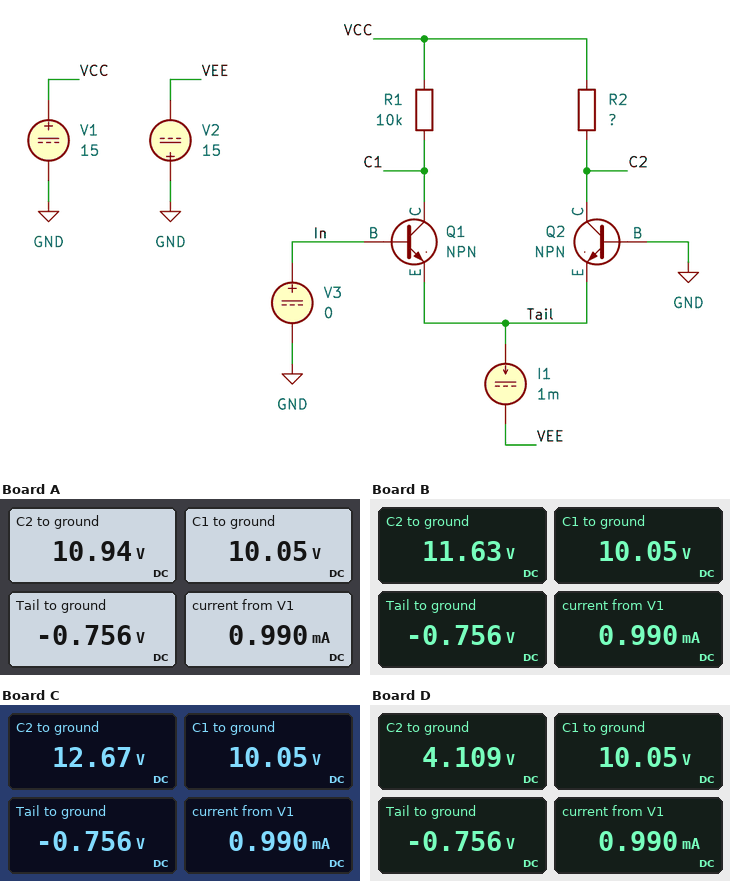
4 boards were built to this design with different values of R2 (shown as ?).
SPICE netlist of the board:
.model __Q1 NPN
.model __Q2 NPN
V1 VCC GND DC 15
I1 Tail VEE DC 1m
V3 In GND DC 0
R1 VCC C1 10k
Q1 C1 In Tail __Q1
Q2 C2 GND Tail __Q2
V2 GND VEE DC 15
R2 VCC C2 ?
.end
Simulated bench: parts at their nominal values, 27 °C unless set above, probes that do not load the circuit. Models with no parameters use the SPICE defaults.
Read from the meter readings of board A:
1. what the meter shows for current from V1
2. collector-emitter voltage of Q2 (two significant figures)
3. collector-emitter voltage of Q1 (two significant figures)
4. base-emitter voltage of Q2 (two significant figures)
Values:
0.990 mA
12 V
11 V
760 mV
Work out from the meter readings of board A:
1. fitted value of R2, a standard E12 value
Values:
8.2 kΩ
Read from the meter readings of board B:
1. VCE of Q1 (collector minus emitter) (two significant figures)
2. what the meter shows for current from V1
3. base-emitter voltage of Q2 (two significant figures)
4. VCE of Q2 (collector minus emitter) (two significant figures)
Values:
11 V
0.990 mA
760 mV
12 V
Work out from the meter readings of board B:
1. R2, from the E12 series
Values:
6.8 kΩ
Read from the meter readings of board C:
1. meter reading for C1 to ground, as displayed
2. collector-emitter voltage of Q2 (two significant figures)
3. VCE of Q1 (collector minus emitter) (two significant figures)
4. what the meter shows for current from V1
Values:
10.05 V
13 V
11 V
0.990 mA
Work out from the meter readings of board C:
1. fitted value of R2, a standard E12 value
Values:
4.7 kΩ
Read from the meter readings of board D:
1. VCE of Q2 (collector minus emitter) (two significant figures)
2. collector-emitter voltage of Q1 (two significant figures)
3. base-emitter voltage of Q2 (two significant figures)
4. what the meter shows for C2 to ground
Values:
4.9 V
11 V
760 mV
4.109 V
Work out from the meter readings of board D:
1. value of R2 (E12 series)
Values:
22 kΩ
